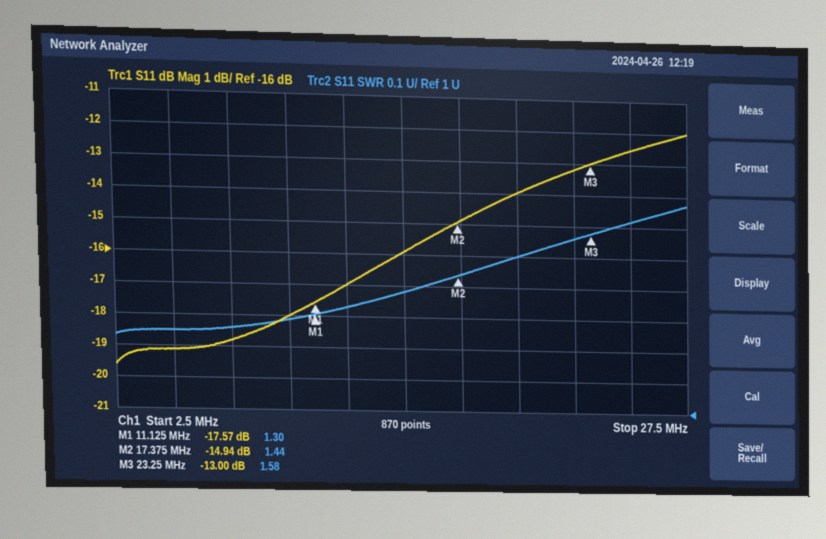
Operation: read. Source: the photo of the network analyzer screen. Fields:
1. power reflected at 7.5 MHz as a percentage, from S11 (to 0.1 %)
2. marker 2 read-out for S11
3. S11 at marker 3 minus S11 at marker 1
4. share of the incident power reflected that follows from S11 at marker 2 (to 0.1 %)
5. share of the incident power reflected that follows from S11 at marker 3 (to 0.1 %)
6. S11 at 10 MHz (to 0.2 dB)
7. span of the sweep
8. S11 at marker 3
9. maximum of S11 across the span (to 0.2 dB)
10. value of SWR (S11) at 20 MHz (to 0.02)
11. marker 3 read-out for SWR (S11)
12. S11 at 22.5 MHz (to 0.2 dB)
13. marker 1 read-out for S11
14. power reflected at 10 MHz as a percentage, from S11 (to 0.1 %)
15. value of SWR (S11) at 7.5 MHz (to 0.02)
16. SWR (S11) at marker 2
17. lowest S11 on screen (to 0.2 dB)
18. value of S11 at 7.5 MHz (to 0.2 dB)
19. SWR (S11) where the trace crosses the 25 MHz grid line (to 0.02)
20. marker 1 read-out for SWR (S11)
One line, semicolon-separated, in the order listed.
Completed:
1.3 %; -14.94 dB; 4.57 dB; 3.2 %; 5.0 %; -18.0 dB; 25 MHz; -13.00 dB; -12.0 dB; 1.50; 1.58; -13.2 dB; -17.57 dB; 1.6 %; 1.26; 1.44; -19.6 dB; -18.8 dB; 1.62; 1.30
